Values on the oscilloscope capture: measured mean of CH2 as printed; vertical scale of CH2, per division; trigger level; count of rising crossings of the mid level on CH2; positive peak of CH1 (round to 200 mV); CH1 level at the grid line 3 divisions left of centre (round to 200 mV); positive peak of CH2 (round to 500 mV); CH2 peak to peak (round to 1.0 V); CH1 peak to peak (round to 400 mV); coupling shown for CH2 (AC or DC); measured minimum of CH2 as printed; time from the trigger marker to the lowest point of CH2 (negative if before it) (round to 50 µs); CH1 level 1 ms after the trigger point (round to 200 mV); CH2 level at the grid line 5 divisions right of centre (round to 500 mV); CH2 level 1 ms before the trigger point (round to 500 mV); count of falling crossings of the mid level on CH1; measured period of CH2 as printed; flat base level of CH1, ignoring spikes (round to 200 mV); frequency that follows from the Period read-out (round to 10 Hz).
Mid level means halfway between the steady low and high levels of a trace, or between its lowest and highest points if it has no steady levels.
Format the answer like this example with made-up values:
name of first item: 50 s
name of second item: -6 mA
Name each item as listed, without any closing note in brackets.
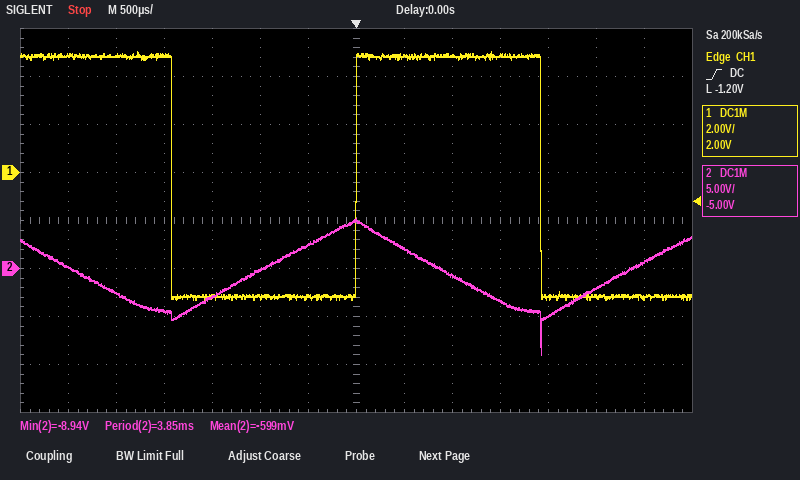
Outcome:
measured mean of CH2 as printed: -599 mV
vertical scale of CH2, per division: 5 V
trigger level: -1.20 V
count of rising crossings of the mid level on CH2: 2
positive peak of CH1: 5.0 V
CH1 level at the grid line 3 divisions left of centre: -5.2 V
positive peak of CH2: 5.0 V
CH2 peak to peak: 14.0 V
CH1 peak to peak: 10.4 V
coupling shown for CH2: DC
measured minimum of CH2 as printed: -8.94 V
time from the trigger marker to the lowest point of CH2 (negative if before it): +1.95 ms
CH1 level 1 ms after the trigger point: 4.8 V
CH2 level at the grid line 5 divisions right of centre: -2.0 V
CH2 level 1 ms before the trigger point: 0.0 V
count of falling crossings of the mid level on CH1: 2
measured period of CH2 as printed: 3.85 ms
flat base level of CH1, ignoring spikes: -5.2 V
frequency that follows from the Period read-out: 260 Hz
